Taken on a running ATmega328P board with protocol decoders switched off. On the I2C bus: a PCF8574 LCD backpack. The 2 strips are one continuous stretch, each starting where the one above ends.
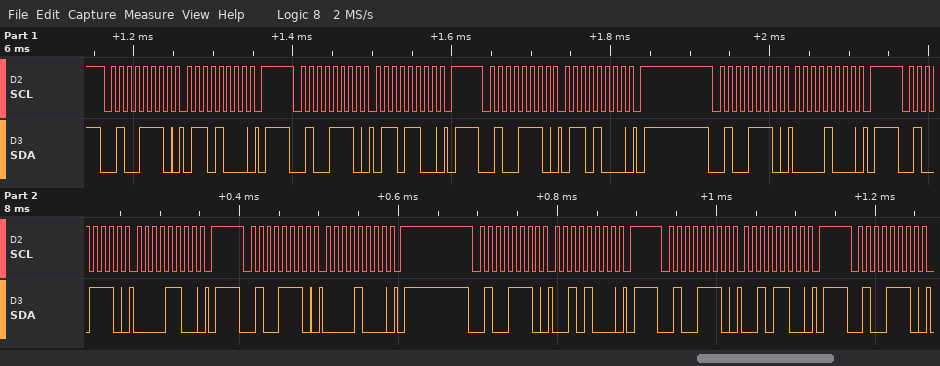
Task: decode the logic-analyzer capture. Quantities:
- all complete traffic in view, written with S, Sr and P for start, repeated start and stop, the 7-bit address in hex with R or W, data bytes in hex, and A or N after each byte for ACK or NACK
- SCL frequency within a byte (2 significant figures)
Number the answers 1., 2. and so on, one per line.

1. S 27W A 68 A P S 27W A 6C A P S 27W A 68 A P S 27W A 08 A P S 27W A 0C A P S 27W A 08 A P S 27W A 28 A P S 27W A 2C A P S 27W A
2. 100 kHz
